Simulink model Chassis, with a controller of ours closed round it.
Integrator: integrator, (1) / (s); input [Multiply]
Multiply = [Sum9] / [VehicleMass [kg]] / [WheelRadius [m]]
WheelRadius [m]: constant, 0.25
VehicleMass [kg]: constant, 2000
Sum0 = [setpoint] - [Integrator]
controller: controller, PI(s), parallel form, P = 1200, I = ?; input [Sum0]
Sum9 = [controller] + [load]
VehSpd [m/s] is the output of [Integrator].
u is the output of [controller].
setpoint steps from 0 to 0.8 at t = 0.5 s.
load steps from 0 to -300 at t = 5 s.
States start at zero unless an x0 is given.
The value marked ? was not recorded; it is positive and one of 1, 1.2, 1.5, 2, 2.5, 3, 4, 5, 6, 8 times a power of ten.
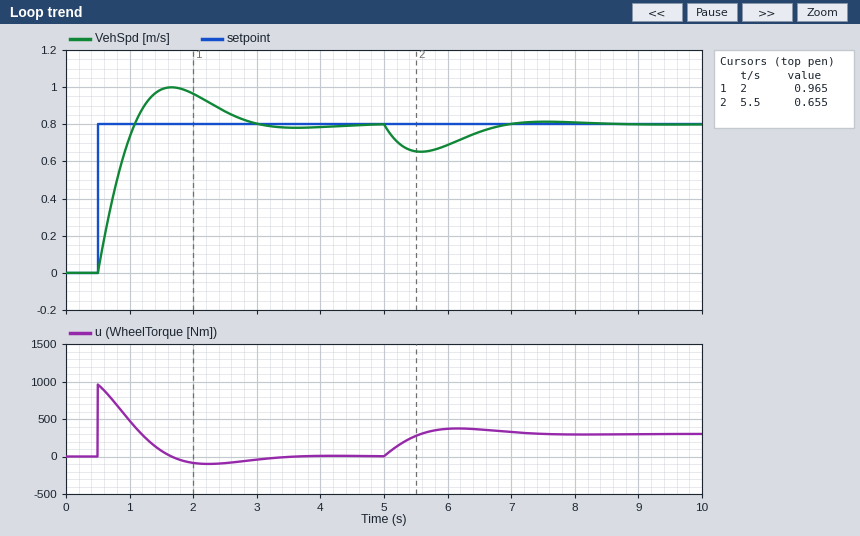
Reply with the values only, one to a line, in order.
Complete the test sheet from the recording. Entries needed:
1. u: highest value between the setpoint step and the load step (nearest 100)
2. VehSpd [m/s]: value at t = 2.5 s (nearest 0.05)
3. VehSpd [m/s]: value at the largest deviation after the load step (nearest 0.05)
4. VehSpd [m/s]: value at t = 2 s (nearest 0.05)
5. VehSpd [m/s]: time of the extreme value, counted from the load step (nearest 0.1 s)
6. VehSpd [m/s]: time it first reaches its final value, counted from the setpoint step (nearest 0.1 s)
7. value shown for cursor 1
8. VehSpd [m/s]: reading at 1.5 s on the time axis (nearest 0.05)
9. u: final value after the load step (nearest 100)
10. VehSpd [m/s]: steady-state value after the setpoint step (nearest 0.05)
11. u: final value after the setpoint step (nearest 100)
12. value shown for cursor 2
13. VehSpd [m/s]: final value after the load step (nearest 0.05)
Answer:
1000
0.85
0.65
0.95
0.6 s
0.6 s
0.965
1.00
300
0.80
0
0.655
0.80
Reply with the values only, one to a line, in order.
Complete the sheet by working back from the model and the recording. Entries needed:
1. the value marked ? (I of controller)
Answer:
2000
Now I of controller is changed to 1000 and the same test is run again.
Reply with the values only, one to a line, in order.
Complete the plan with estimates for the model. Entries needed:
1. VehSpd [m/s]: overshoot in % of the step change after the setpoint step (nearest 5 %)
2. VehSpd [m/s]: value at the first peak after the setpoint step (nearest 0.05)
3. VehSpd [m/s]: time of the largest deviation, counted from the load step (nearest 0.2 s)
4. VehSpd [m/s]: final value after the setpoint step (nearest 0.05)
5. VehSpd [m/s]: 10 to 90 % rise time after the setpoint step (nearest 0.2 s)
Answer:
15 %
0.95
0.8 s
0.80
0.6 s
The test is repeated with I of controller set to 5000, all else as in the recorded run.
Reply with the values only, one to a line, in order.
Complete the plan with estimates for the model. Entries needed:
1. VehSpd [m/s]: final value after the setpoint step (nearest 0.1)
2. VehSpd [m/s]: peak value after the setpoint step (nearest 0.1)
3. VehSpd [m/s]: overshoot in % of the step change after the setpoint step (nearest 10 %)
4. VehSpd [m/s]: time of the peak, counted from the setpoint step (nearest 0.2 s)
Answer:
0.8
1.1
40 %
0.8 s
